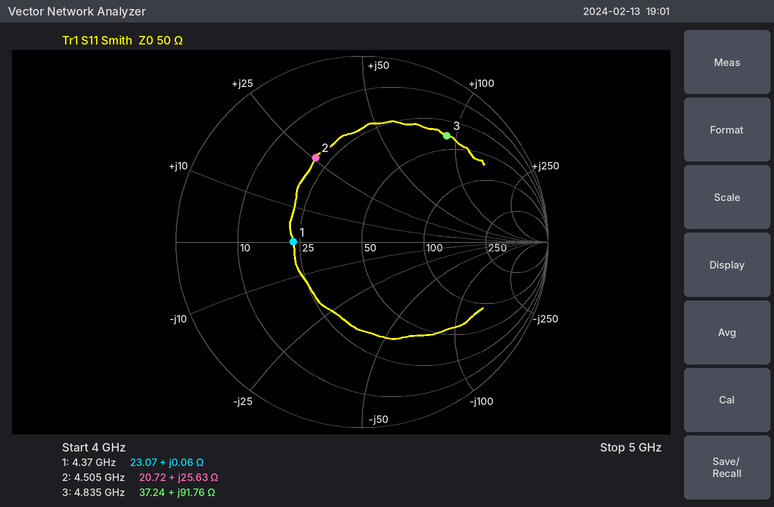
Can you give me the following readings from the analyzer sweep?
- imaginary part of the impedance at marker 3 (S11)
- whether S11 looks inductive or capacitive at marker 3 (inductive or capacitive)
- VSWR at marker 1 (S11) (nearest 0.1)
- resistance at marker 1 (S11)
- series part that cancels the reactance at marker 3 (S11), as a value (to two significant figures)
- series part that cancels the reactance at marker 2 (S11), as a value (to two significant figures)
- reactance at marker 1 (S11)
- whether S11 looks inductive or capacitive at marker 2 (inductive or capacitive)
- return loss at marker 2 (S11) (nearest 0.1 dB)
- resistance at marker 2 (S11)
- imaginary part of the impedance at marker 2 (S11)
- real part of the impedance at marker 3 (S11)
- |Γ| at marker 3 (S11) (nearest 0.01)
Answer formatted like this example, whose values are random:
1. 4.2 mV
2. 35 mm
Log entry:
1. +91.76 Ω
2. inductive
3. 2.2
4. 23.07 Ω
5. 360 fF
6. 1.4 pF
7. +0.06 Ω
8. inductive
9. 5.7 dB
10. 20.72 Ω
11. +25.63 Ω
12. 37.24 Ω
13. 0.73
